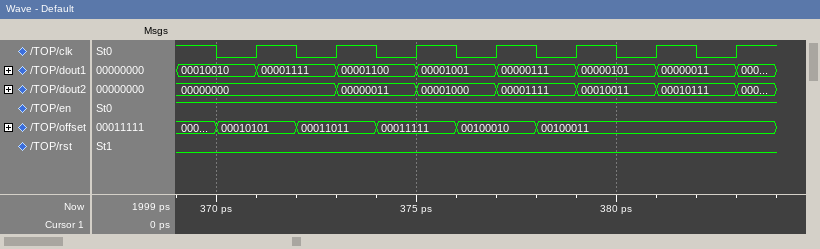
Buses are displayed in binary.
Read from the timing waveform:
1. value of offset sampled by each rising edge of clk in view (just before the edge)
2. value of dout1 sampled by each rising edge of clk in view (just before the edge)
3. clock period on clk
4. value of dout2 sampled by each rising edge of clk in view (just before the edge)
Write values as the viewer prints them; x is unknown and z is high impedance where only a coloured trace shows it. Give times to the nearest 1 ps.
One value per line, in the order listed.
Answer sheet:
00010101, 00011011, 00011111, 00100010, 00100011, 00100011, 00100011
00010010, 00001111, 00001100, 00001001, 00000111, 00000101, 00000011
2 ps
00000000, 00000000, 00000011, 00001000, 00001111, 00010011, 00010111
